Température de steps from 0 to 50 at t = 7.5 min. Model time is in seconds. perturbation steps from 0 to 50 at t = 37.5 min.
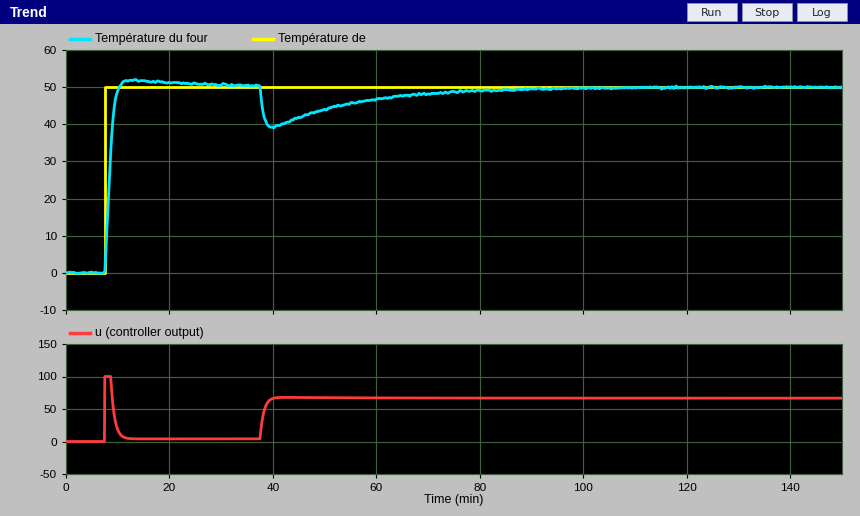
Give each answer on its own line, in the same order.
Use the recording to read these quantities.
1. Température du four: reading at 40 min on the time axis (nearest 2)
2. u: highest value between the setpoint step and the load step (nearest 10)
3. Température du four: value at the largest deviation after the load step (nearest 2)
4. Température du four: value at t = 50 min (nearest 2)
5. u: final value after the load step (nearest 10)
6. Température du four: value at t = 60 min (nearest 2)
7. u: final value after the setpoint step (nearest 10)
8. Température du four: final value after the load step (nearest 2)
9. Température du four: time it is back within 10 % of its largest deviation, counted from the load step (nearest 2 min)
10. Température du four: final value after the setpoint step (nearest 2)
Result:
40
100
40
44
70
46
0
50
40 min
50
